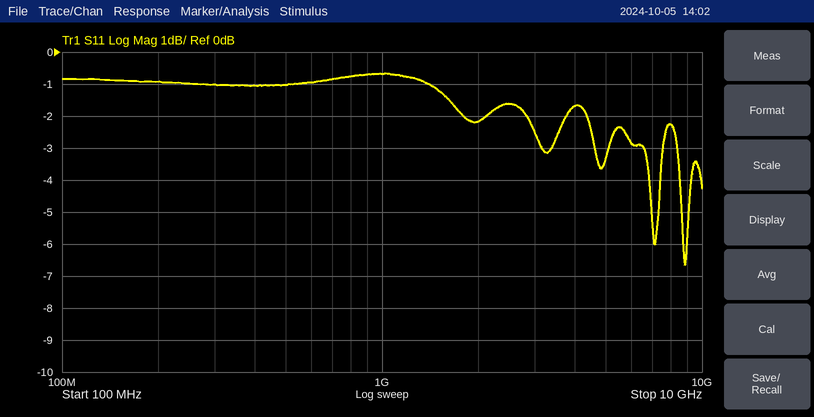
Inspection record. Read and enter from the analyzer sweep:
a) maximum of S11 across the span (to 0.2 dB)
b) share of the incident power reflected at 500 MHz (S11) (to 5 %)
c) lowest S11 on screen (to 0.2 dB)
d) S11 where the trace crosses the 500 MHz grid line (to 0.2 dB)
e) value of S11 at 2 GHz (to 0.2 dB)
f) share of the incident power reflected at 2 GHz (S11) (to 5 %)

-0.6 dB
80 %
-6.6 dB
-1.0 dB
-2.2 dB
60 %
